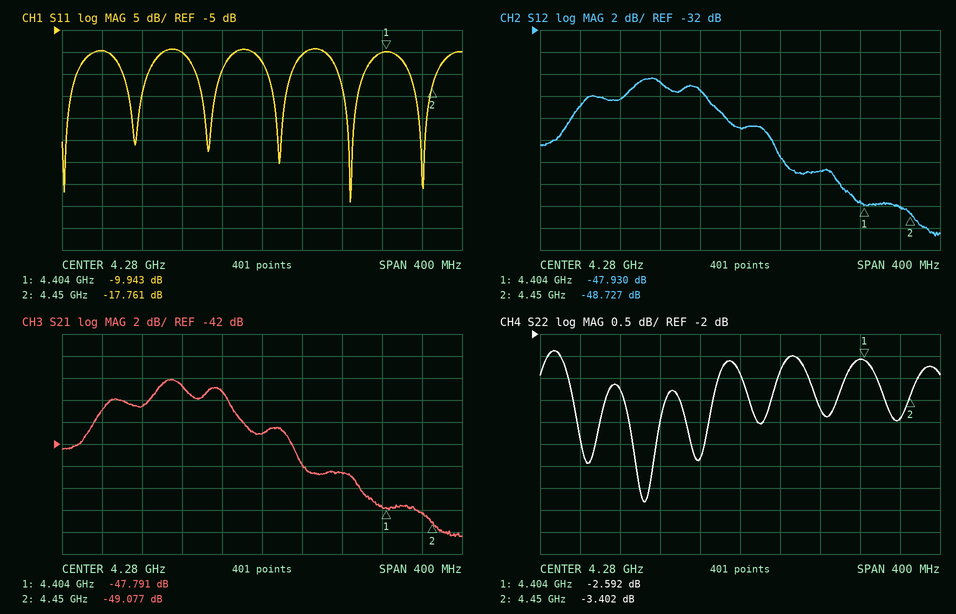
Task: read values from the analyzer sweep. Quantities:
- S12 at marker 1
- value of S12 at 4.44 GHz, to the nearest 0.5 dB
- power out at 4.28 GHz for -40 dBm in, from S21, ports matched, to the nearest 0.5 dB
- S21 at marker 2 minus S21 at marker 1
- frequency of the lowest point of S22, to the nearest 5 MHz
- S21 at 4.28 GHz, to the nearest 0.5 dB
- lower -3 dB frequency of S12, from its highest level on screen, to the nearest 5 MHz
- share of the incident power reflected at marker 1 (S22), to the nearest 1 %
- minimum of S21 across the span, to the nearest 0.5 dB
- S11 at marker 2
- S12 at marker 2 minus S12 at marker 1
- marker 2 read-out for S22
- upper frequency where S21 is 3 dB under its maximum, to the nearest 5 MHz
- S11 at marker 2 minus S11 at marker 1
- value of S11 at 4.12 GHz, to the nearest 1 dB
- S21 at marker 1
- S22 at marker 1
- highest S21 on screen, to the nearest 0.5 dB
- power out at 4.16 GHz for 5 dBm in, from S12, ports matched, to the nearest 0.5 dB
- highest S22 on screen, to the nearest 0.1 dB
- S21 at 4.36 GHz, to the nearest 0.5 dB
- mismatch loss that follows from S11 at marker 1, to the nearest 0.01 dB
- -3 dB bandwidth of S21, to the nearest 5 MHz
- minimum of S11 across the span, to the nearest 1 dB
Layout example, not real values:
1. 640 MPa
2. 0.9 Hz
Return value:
1. -47.930 dB
2. -48.0 dB
3. -81.0 dBm
4. -1.286 dB
5. 4.185 GHz
6. -41.0 dB
7. 4.115 GHz
8. 55 %
9. -50.5 dB
10. -17.761 dB
11. -0.797 dB
12. -3.402 dB
13. 4.255 GHz
14. -7.818 dB
15. -10 dB
16. -47.791 dB
17. -2.592 dB
18. -36.0 dB
19. -33.5 dBm
20. -2.4 dB
21. -44.5 dB
22. 0.46 dB
23. 135 MHz
24. -44 dB
